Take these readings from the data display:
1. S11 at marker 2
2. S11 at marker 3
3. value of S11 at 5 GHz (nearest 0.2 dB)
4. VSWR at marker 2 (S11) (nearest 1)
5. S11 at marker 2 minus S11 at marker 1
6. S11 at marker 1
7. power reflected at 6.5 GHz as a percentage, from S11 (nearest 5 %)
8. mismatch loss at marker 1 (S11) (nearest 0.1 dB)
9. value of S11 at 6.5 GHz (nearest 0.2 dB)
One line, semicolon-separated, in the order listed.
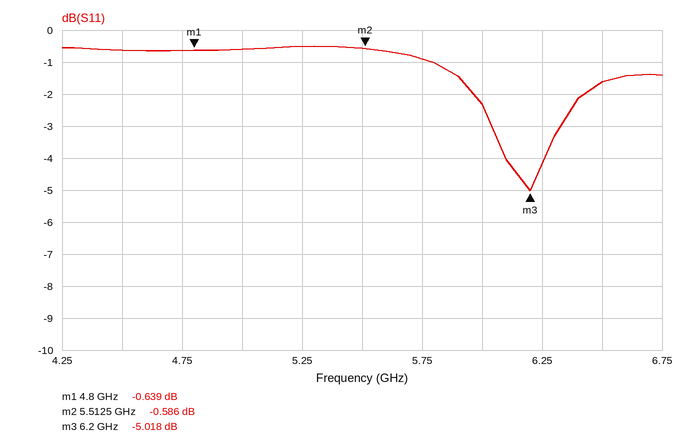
-0.586 dB; -5.018 dB; -0.6 dB; 30; 0.053 dB; -0.639 dB; 70 %; 8.6 dB; -1.6 dB
